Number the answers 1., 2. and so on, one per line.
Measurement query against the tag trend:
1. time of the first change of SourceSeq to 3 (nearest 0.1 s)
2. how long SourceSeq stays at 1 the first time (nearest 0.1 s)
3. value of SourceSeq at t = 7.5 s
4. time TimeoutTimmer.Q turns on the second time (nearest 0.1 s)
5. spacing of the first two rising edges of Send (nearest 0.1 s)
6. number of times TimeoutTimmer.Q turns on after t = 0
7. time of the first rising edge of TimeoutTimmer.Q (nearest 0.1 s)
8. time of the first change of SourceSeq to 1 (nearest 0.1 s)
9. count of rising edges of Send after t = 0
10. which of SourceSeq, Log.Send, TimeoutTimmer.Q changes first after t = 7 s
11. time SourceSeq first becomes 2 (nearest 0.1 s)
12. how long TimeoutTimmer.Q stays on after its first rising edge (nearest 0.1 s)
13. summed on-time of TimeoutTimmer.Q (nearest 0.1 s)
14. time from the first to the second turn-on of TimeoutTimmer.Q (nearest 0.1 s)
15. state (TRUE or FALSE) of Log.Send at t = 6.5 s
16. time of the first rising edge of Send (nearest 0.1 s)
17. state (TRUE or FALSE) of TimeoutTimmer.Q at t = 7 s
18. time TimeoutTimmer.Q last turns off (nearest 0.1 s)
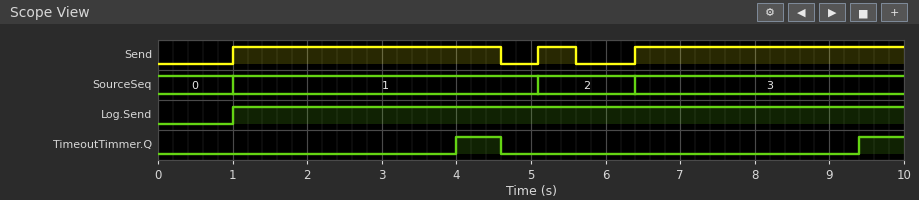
1. 6.4 s
2. 4.1 s
3. 3
4. 9.4 s
5. 4.1 s
6. 2
7. 4.0 s
8. 1.0 s
9. 3
10. TimeoutTimmer.Q
11. 5.1 s
12. 0.6 s
13. 1.2 s
14. 5.4 s
15. TRUE
16. 1.0 s
17. FALSE
18. 4.6 s
